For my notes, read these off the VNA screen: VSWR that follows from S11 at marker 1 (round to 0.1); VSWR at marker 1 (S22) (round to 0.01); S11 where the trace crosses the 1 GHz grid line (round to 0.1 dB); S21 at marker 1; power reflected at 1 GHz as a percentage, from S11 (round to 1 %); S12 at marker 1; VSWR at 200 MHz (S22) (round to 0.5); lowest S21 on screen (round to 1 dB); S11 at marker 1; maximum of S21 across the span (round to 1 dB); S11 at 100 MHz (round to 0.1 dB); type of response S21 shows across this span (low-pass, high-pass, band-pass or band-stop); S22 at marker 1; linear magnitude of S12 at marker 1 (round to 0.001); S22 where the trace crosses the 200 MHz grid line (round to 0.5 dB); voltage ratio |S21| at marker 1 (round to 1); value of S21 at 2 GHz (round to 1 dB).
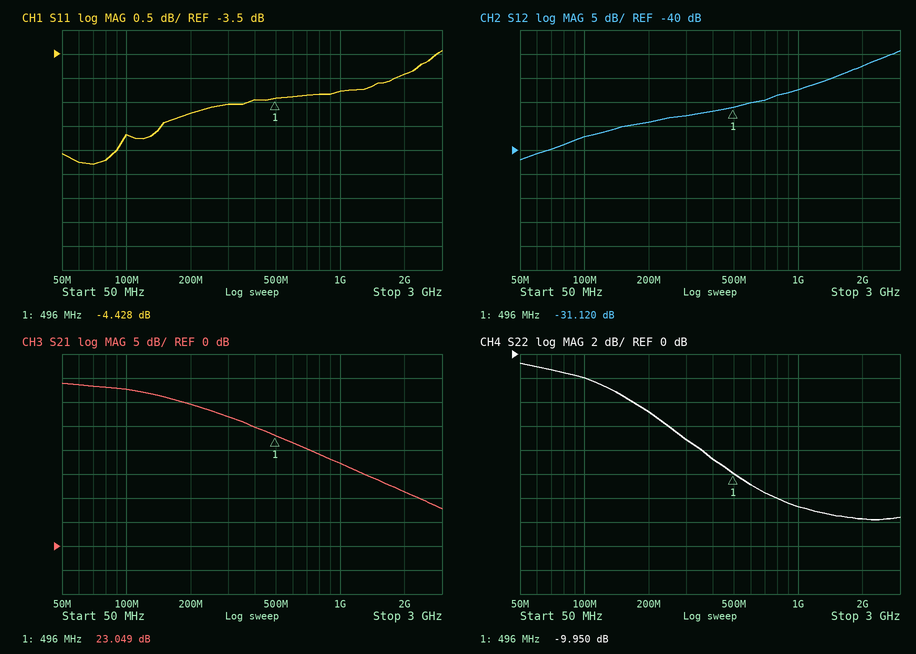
4.0
1.93
-4.3 dB
23.049 dB
37 %
-31.120 dB
3.5
8 dB
-4.428 dB
34 dB
-5.2 dB
low-pass
-9.950 dB
0.028
-5.0 dB
14
11 dB
